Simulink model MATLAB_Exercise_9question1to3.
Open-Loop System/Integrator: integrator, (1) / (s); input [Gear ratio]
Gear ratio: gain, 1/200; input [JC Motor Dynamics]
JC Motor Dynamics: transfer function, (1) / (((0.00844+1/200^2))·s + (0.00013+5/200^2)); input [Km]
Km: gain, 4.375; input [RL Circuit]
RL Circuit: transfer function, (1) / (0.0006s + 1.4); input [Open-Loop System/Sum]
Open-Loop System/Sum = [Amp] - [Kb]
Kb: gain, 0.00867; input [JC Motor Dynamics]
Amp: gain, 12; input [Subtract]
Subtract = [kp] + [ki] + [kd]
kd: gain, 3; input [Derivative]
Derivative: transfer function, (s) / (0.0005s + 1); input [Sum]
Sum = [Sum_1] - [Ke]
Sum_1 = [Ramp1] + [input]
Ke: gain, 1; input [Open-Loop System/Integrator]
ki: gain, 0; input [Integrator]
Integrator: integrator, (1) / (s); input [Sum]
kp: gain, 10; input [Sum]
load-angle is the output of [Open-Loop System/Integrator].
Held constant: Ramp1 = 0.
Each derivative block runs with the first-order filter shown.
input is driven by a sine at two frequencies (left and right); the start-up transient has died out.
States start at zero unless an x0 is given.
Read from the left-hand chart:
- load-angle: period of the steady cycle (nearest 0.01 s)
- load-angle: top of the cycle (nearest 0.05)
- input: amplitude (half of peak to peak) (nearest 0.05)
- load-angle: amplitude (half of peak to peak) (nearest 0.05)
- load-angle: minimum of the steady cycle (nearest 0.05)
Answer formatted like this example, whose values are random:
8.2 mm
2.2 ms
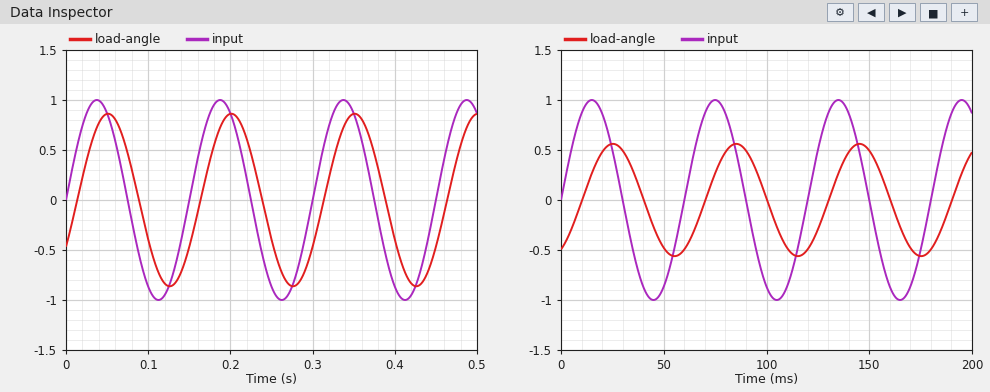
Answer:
0.15 s
0.85
1.00
0.85
-0.85
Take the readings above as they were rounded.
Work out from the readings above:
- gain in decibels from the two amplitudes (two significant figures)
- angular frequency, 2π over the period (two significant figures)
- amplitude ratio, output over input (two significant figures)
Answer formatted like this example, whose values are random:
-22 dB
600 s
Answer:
-1.4 dB
42 rad/s
0.85
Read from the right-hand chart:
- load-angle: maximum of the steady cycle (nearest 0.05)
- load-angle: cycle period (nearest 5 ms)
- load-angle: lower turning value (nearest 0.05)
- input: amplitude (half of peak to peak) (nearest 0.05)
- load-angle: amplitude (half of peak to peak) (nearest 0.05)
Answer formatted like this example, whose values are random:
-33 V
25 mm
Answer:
0.55
60 ms
-0.55
1.00
0.55
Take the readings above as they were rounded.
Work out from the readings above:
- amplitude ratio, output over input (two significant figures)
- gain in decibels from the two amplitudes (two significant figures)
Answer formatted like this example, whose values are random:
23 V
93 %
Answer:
0.55
-5.2 dB
